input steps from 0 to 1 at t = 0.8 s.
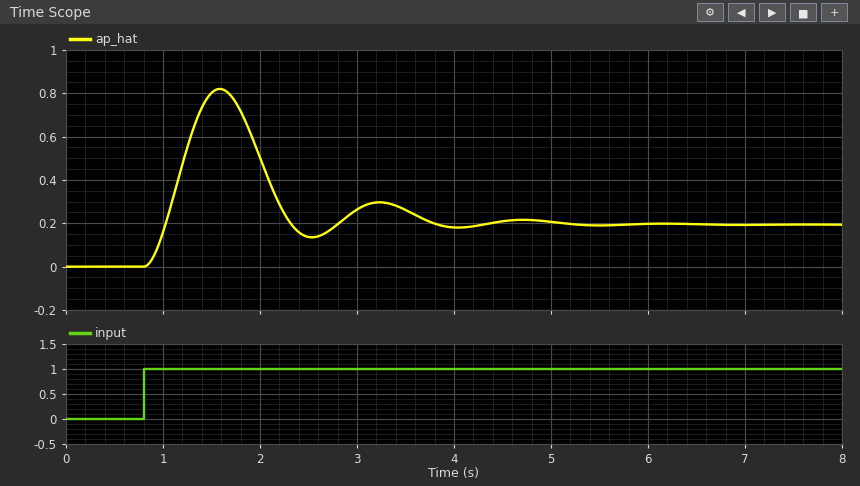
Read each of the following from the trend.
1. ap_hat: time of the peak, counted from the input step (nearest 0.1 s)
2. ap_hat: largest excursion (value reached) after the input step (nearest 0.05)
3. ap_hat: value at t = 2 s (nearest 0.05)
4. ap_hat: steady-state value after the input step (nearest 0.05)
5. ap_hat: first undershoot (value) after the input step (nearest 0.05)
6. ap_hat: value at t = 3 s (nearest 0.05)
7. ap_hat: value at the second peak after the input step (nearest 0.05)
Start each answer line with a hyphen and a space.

- 0.8 s
- 0.80
- 0.50
- 0.20
- 0.15
- 0.25
- 0.30
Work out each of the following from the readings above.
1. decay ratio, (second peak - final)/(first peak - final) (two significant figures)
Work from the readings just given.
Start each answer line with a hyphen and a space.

- 0.17
